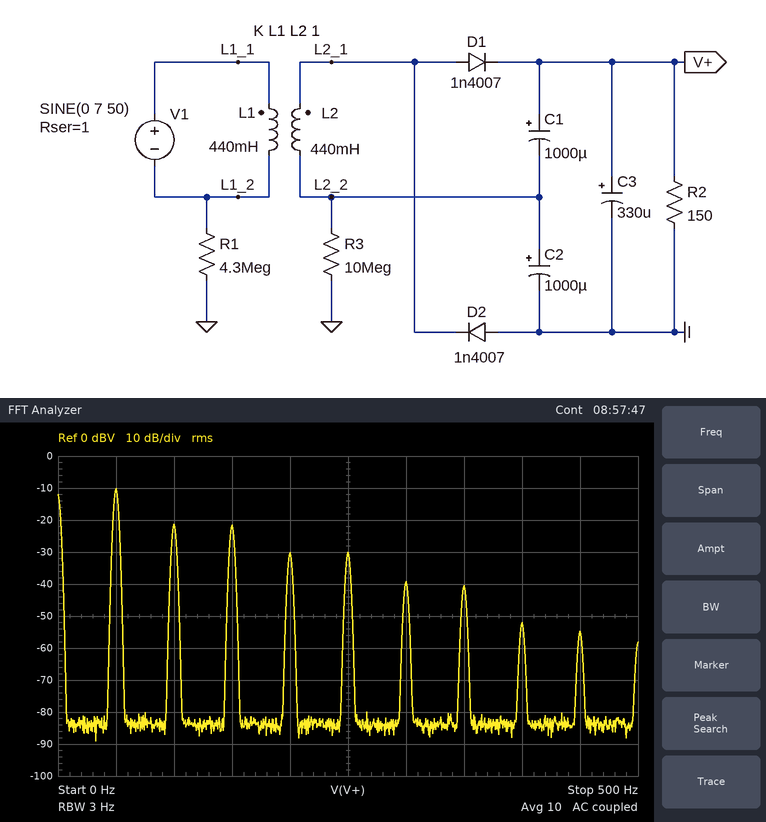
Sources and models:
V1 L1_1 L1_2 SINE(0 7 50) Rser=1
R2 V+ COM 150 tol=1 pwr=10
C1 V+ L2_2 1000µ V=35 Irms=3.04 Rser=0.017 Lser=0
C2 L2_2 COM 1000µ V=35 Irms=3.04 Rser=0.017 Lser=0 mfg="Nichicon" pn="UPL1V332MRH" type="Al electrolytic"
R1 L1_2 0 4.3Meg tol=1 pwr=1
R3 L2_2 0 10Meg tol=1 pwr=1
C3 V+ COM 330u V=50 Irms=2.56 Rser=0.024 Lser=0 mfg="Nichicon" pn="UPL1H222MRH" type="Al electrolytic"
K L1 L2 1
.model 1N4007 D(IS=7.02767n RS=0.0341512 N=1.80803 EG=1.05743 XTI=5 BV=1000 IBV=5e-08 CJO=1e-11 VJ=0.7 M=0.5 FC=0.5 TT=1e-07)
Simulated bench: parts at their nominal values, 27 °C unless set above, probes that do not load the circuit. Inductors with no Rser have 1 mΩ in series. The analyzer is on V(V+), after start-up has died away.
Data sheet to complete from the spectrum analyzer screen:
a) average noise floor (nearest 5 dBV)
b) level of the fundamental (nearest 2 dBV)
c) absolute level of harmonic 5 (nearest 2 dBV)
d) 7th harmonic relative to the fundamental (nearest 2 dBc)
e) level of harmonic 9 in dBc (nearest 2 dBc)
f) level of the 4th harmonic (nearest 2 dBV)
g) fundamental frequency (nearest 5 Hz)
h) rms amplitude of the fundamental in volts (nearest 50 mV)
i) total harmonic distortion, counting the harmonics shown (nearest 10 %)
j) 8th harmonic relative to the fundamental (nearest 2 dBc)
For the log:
-85 dBV
-10 dBV
-30 dBV
-30 dBc
-44 dBc
-30 dBV
50 Hz
300 mV
40 %
-42 dBc
